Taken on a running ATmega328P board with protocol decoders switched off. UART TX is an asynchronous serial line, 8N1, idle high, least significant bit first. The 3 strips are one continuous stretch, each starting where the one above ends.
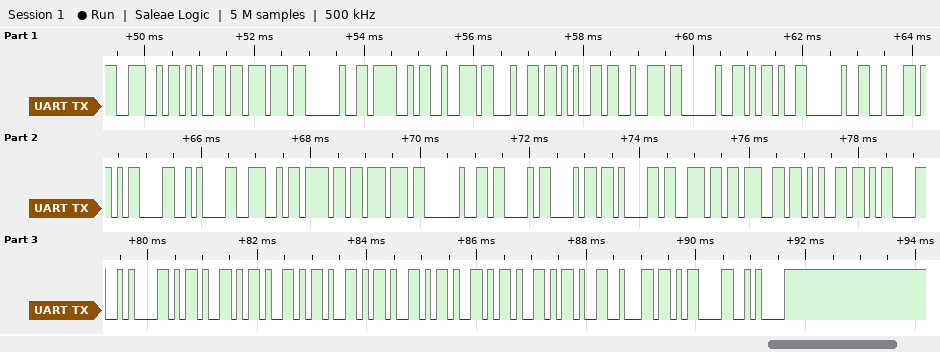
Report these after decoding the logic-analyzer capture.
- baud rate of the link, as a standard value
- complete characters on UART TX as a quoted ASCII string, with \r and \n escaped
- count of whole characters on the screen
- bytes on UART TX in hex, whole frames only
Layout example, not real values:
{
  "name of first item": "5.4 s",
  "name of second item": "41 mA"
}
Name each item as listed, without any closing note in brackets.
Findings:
{
  "baud rate of the link, as a standard value": "9600 baud",
  "complete characters on UART TX as a quoted ASCII string, with \\r and \\n escaped": "\"New Order - b\\r\\nNow Change\\r\\n-------b\\r\\n\"",
  "count of whole characters on the screen": "37",
  "bytes on UART TX in hex, whole frames only": "0x4E 0x65 0x77 0x20 0x4F 0x72 0x64 0x65 0x72 0x20 0x2D 0x20 0x62 0x0D 0x0A 0x4E 0x6F 0x77 0x20 0x43 0x68 0x61 0x6E 0x67 0x65 0x0D 0x0A 0x2D 0x2D 0x2D 0x2D 0x2D 0x2D 0x2D 0x62 0x0D 0x0A"
}
